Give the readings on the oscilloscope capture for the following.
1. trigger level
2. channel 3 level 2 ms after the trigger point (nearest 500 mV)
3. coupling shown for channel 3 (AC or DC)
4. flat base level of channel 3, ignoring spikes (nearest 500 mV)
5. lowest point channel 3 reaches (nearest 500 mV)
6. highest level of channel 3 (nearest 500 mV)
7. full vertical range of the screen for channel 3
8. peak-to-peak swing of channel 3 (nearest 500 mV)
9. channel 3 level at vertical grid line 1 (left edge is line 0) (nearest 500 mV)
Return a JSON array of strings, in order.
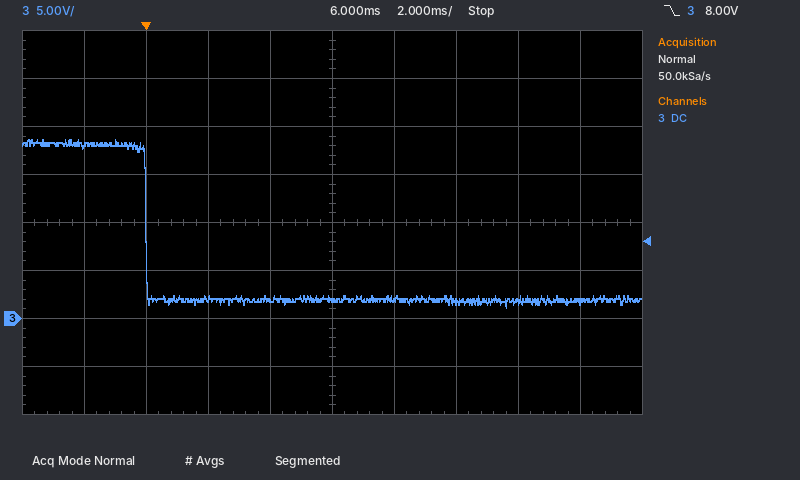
["8.00 V", "2.0 V", "DC", "2.0 V", "1.0 V", "18.5 V", "40 V", "17.5 V", "18.0 V"]
